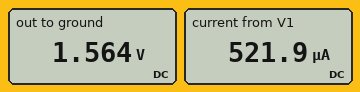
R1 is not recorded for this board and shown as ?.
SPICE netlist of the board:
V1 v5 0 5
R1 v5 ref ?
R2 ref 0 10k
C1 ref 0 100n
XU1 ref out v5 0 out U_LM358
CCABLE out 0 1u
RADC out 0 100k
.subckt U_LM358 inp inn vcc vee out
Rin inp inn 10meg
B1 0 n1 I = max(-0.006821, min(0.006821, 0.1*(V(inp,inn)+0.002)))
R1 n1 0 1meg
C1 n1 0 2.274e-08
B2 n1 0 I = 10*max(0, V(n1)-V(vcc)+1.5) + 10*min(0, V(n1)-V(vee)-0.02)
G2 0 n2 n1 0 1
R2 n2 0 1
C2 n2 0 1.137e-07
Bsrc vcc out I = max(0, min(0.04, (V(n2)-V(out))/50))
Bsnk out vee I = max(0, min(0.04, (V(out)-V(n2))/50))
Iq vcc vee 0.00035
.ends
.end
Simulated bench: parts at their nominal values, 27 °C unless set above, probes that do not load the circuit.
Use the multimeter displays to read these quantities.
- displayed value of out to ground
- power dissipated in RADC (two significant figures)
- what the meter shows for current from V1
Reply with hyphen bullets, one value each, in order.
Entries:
- 1.564 V
- 24 µW
- 521.9 µA
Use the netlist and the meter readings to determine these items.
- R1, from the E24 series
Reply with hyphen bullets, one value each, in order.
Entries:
- 22 kΩ
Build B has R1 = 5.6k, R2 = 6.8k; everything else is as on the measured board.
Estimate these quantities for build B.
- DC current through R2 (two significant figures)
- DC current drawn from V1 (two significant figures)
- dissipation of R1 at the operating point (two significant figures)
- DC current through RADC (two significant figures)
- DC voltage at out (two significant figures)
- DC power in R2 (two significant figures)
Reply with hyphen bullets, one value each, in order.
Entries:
- 400 µA
- 780 µA
- 910 µW
- 27 µA
- 2.7 V
- 1.1 mW
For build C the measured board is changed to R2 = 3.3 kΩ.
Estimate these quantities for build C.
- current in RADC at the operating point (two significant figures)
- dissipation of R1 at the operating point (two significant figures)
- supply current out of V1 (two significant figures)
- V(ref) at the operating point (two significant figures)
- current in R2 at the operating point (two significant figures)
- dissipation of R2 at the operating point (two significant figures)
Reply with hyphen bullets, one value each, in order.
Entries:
- 6.5 µA
- 860 µW
- 550 µA
- 650 mV
- 200 µA
- 130 µW
